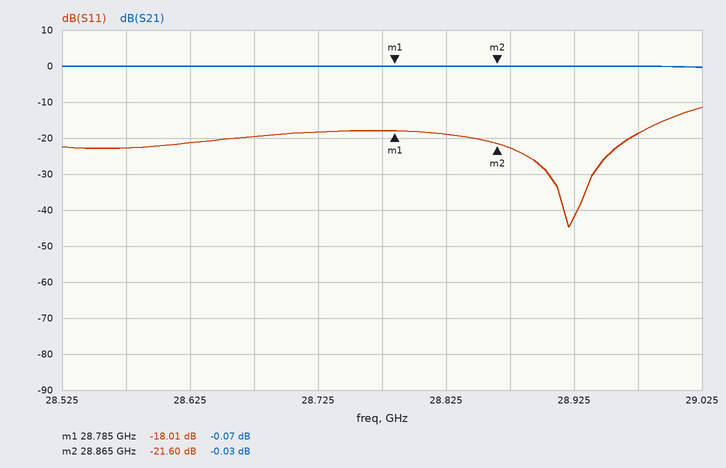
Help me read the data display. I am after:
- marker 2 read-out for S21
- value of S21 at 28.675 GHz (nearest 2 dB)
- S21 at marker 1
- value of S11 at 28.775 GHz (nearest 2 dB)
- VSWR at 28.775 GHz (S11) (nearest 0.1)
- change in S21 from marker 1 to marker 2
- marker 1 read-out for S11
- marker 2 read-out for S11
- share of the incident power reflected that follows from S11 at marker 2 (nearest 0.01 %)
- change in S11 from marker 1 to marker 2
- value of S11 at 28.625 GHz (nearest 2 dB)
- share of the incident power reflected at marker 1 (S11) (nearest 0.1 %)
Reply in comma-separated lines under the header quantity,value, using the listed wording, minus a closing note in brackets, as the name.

quantity,value
marker 2 read-out for S21,-0.03 dB
value of S21 at 28.675 GHz,0 dB
S21 at marker 1,-0.07 dB
value of S11 at 28.775 GHz,-18 dB
VSWR at 28.775 GHz (S11),1.3
change in S21 from marker 1 to marker 2,0.04 dB
marker 1 read-out for S11,-18.01 dB
marker 2 read-out for S11,-21.60 dB
share of the incident power reflected that follows from S11 at marker 2,0.69 %
change in S11 from marker 1 to marker 2,-3.59 dB
value of S11 at 28.625 GHz,-22 dB
share of the incident power reflected at marker 1 (S11),1.6 %
